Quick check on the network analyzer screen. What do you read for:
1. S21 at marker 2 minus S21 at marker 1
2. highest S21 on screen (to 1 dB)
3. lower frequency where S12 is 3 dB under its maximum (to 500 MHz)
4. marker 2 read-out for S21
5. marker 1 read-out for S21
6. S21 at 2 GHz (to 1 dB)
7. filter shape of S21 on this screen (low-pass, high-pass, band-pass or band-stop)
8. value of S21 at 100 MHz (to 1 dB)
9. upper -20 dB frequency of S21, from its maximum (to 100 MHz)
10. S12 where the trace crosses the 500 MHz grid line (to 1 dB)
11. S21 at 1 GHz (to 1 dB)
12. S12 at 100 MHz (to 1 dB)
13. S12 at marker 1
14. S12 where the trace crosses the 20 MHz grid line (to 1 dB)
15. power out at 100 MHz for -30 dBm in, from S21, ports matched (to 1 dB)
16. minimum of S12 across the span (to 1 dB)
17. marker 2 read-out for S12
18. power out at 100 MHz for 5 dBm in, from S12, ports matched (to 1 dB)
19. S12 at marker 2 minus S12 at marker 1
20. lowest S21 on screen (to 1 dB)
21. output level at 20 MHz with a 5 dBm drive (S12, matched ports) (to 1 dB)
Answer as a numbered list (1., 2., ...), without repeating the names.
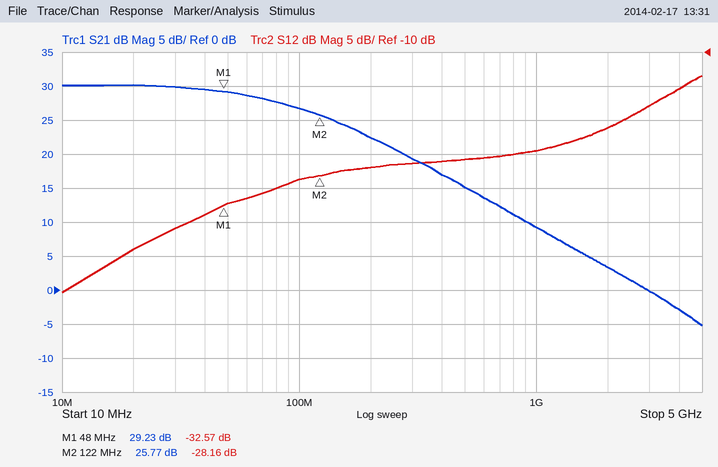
1. -3.46 dB
2. 30 dB
3. 3.5 GHz
4. 25.77 dB
5. 29.23 dB
6. 3 dB
7. low-pass
8. 27 dB
9. 900 MHz
10. -26 dB
11. 9 dB
12. -29 dB
13. -32.57 dB
14. -39 dB
15. -3 dBm
16. -45 dB
17. -28.16 dB
18. -24 dBm
19. 4.41 dB
20. -5 dB
21. -34 dBm
